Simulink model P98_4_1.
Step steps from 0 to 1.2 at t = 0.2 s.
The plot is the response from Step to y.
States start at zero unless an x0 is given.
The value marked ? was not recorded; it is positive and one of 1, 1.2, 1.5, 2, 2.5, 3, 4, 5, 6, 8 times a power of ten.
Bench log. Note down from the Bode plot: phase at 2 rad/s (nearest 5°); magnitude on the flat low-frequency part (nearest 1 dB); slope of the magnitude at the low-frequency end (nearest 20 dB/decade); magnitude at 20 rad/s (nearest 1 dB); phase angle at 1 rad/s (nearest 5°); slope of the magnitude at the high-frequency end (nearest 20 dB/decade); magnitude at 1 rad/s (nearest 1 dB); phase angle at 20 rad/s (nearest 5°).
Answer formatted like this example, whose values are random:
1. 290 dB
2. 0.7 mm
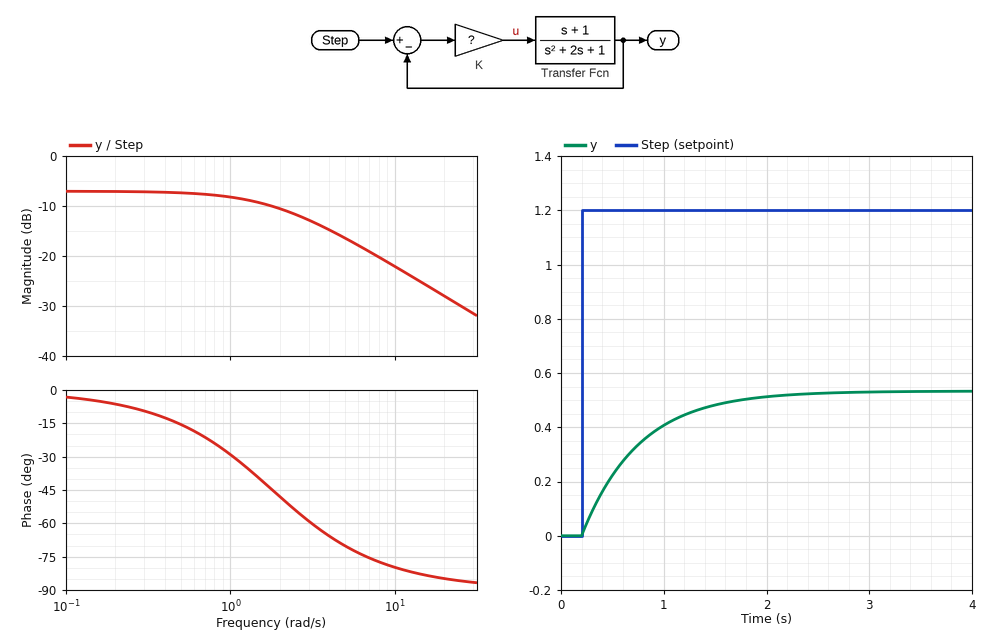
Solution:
1. -50°
2. -7 dB
3. 0 dB/decade
4. -28 dB
5. -30°
6. -20 dB/decade
7. -8 dB
8. -85°
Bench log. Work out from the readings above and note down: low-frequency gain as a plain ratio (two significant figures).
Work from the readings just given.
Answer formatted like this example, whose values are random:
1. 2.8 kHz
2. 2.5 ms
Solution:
1. 0.45
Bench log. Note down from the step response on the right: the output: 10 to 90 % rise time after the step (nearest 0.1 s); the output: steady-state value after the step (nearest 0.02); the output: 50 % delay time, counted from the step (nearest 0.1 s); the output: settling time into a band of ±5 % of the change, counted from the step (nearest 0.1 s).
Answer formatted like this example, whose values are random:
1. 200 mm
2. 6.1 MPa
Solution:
1. 1.2 s
2. 0.54
3. 0.4 s
4. 1.7 s
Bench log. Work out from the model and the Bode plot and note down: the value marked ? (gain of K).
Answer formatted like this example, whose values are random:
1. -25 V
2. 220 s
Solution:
1. 0.8
